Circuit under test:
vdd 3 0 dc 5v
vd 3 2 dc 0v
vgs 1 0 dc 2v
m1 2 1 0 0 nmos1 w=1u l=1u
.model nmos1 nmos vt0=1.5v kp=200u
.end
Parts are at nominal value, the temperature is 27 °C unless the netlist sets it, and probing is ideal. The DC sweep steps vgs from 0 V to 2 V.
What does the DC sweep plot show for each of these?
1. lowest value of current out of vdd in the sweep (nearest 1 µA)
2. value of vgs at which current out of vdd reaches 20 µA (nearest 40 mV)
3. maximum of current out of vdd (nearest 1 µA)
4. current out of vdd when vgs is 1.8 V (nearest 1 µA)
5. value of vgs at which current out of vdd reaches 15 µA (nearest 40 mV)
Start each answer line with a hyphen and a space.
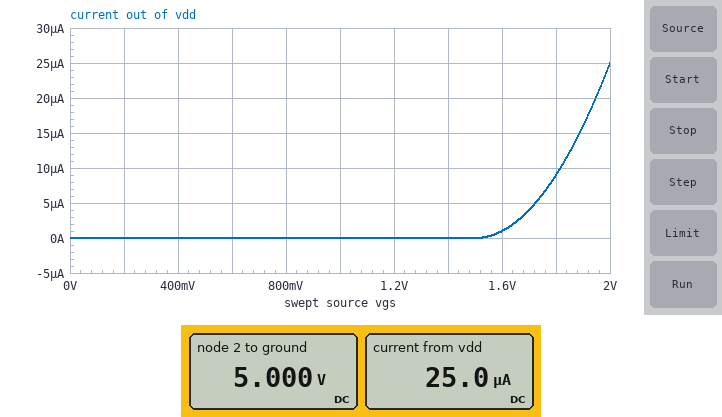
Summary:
- 0 A
- 1.96 V
- 25 µA
- 9 µA
- 1.88 V
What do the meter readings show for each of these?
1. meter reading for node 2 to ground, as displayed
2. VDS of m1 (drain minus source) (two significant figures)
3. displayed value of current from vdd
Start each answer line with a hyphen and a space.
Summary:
- 5.000 V
- 5.0 V
- 25.0 µA
